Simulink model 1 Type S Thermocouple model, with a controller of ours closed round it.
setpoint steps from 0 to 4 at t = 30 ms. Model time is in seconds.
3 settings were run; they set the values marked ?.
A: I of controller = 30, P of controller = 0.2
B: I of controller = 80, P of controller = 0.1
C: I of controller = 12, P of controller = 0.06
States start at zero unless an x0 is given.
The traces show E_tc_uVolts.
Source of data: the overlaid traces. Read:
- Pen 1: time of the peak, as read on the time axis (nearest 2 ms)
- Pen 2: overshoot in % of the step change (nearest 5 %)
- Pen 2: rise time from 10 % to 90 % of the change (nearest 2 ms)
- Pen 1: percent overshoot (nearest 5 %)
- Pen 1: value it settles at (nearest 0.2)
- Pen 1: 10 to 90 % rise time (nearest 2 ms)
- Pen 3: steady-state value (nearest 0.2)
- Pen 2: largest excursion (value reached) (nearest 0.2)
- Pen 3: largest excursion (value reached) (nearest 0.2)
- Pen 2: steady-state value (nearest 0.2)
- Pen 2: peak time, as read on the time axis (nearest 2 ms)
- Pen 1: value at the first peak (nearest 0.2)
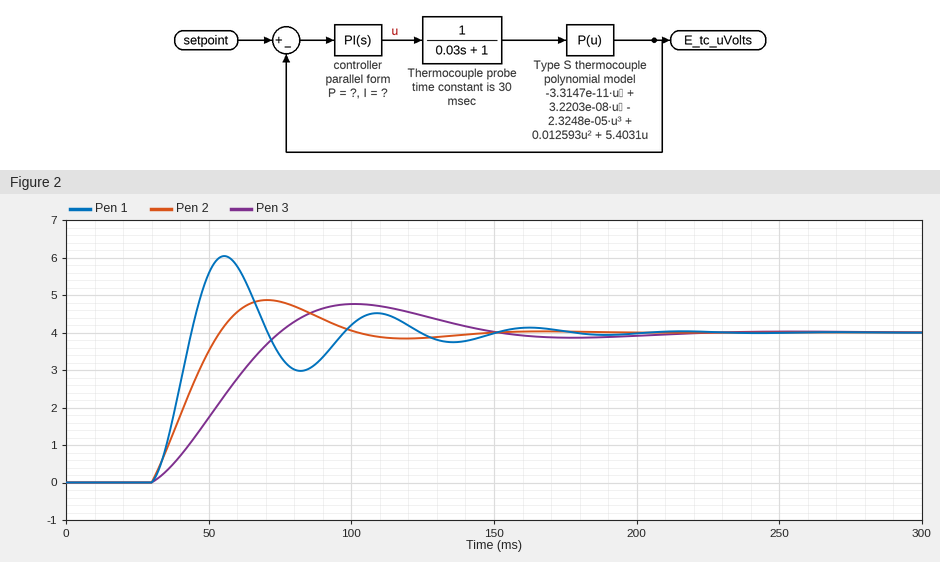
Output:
56 ms
20 %
18 ms
50 %
4.0
10 ms
4.0
4.8
4.8
4.0
70 ms
6.0
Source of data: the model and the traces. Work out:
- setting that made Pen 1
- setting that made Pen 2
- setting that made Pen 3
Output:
B
A
C
